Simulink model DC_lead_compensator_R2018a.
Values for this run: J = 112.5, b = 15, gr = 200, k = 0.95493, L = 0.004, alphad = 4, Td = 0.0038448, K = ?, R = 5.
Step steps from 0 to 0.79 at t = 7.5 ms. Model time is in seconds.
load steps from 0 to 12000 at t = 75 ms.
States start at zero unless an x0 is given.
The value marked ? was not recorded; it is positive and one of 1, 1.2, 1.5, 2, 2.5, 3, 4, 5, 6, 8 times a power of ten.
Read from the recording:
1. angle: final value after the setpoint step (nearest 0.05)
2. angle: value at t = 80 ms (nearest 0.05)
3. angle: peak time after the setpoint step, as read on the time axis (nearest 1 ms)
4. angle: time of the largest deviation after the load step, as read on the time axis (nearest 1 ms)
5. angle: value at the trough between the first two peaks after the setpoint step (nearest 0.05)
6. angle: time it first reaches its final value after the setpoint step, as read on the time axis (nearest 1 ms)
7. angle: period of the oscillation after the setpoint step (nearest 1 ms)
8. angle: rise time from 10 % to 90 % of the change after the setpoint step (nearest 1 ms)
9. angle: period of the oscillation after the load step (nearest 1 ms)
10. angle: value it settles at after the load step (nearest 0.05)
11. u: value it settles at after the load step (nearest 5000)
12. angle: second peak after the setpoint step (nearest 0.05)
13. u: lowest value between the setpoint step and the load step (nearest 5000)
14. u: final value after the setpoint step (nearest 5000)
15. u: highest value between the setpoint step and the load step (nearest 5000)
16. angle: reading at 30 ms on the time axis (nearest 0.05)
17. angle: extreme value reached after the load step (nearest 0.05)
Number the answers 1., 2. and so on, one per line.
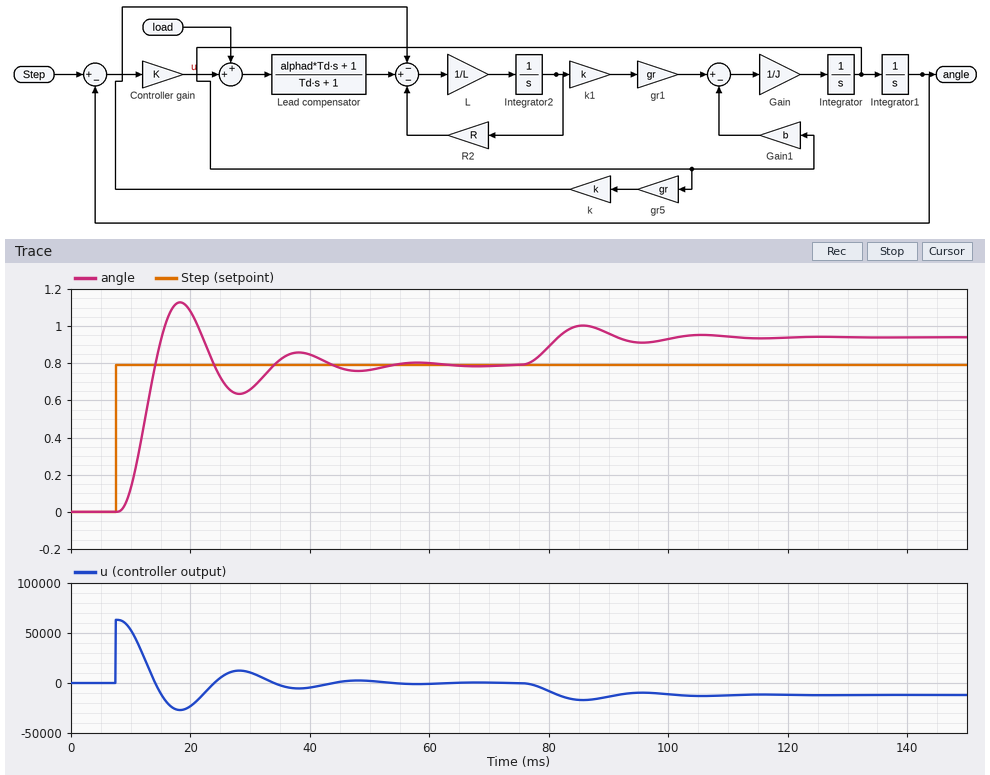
1. 0.80
2. 0.90
3. 18 ms
4. 86 ms
5. 0.65
6. 14 ms
7. 20 ms
8. 4 ms
9. 20 ms
10. 0.95
11. -10000
12. 0.85
13. -25000
14. 0
15. 65000
16. 0.65
17. 1.00
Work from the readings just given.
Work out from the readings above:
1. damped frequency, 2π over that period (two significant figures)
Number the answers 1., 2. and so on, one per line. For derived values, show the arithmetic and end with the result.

1. 2π / 20 = 0.31 rad/ms
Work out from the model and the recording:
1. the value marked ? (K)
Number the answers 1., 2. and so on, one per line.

1. 80000
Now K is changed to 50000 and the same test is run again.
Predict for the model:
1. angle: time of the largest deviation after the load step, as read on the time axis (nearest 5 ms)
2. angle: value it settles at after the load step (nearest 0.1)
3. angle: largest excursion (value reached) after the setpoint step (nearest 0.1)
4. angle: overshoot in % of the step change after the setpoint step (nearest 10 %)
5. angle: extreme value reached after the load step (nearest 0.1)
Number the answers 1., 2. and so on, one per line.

1. 90 ms
2. 1.0
3. 1.0
4. 30 %
5. 1.1
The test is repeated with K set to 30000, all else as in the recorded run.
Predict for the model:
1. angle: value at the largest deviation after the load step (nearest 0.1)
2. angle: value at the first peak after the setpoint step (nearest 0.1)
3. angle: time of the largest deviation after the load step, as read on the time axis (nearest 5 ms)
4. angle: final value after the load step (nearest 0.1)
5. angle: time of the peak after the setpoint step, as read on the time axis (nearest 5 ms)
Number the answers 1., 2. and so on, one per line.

1. 1.2
2. 0.9
3. 95 ms
4. 1.2
5. 25 ms
